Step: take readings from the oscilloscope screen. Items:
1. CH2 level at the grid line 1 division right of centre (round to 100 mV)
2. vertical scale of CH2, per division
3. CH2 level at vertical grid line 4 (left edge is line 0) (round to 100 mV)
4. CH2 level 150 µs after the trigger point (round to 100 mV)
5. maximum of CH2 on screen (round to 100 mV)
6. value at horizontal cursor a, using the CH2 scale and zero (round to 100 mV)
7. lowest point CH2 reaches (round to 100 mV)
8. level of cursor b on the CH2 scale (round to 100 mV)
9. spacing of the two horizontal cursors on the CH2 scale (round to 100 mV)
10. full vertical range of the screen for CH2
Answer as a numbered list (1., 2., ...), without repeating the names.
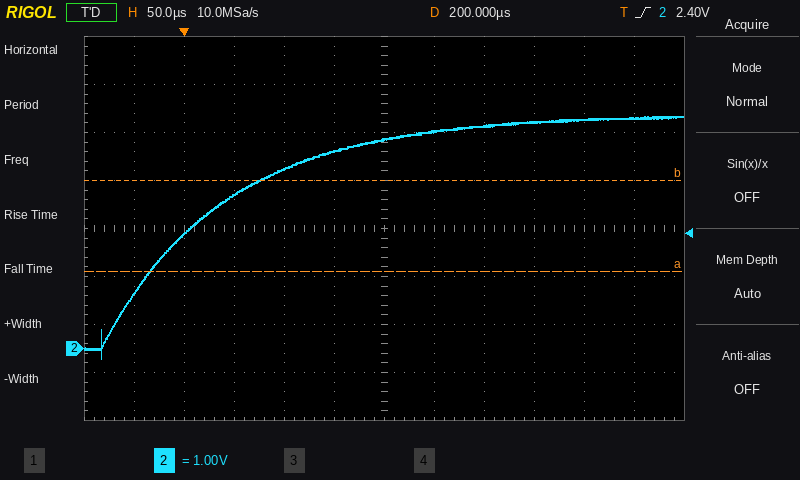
1. 4.5 V
2. 1 V
3. 3.7 V
4. 4.1 V
5. 4.8 V
6. 1.6 V
7. -200 mV
8. 3.5 V
9. 1.9 V
10. 8 V
